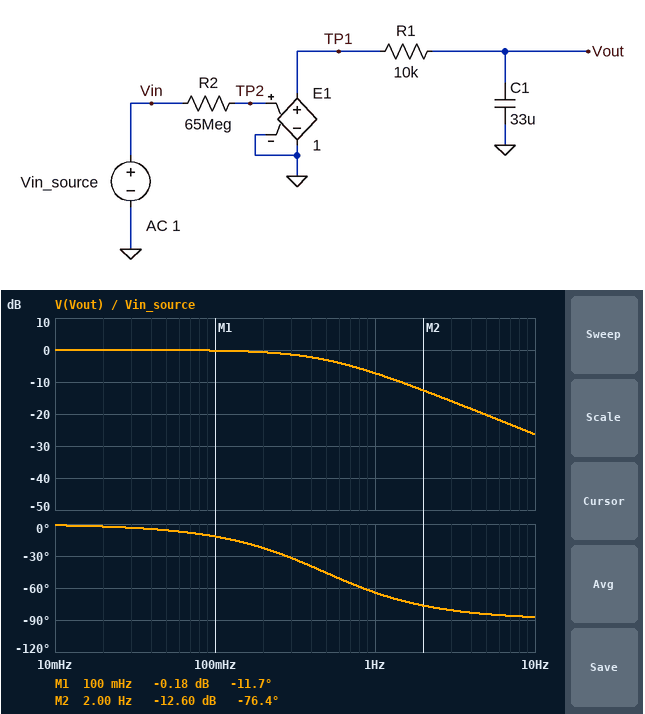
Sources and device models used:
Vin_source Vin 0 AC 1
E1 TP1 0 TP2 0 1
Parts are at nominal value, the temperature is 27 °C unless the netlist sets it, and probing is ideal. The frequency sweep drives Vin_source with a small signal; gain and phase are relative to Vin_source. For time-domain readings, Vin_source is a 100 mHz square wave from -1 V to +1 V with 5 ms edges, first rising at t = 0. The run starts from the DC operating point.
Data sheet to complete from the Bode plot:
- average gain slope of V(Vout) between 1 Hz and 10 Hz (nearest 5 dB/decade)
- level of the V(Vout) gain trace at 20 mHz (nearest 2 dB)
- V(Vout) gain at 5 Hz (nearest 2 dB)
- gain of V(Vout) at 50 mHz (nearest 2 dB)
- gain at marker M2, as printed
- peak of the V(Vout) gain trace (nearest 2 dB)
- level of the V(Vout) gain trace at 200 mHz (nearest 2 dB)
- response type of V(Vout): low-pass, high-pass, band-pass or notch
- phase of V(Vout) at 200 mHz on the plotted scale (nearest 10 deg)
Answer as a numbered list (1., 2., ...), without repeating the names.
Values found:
1. -20 dB/decade
2. 0 dB
3. -20 dB
4. 0 dB
5. -12.60 dB
6. 0 dB
7. 0 dB
8. low-pass
9. -20 deg
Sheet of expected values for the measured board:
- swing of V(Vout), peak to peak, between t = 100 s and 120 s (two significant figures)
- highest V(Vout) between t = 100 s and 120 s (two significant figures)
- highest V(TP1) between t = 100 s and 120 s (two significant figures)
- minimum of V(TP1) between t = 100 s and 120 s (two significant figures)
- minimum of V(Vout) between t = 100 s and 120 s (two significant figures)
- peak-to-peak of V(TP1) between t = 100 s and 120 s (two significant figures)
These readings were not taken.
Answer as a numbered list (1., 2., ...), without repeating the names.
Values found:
1. 2.0 V
2. 1.0 V
3. 1.0 V
4. -1.0 V
5. -1.0 V
6. 2.0 V
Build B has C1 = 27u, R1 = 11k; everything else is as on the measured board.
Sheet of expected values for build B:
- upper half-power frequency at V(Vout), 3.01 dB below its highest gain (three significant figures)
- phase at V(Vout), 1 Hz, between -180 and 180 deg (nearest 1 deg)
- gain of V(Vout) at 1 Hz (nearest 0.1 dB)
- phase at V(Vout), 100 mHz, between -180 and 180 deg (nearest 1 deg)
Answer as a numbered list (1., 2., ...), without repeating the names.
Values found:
1. 536 mHz
2. -62 deg
3. -6.5 dB
4. -11 deg
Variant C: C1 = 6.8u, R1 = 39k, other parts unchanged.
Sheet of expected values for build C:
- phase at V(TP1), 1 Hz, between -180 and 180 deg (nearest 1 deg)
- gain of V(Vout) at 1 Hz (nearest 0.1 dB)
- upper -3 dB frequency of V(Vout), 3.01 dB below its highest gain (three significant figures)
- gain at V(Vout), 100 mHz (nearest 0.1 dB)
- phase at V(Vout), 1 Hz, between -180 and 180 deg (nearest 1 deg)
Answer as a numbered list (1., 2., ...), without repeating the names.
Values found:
1. 0 deg
2. -5.8 dB
3. 600 mHz
4. -0.1 dB
5. -59 deg
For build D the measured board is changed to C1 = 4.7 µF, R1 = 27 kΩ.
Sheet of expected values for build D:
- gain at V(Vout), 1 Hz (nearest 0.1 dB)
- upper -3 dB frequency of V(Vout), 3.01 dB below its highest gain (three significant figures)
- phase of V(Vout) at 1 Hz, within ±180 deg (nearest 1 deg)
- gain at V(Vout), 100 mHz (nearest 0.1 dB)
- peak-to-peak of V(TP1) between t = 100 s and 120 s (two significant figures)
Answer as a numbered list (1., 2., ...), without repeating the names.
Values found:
1. -2.1 dB
2. 1.25 Hz
3. -39 deg
4. 0 dB
5. 2.0 V
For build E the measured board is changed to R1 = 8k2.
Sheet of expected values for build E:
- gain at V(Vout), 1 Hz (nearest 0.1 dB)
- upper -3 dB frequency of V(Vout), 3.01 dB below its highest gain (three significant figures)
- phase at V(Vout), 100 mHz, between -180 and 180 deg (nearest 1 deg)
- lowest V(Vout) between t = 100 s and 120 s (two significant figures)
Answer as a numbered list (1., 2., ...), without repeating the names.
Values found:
1. -5.9 dB
2. 588 mHz
3. -10 deg
4. -1.0 V
